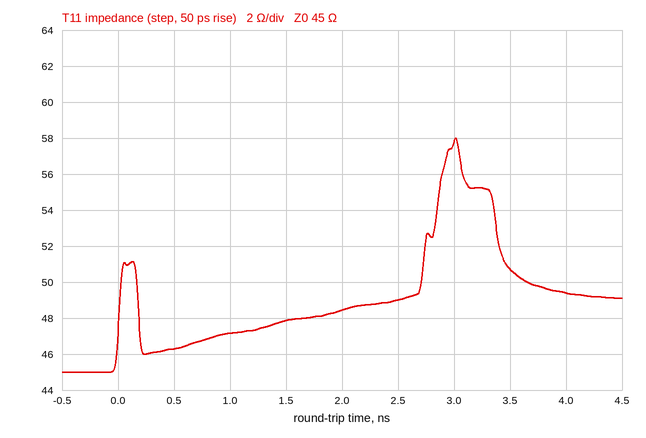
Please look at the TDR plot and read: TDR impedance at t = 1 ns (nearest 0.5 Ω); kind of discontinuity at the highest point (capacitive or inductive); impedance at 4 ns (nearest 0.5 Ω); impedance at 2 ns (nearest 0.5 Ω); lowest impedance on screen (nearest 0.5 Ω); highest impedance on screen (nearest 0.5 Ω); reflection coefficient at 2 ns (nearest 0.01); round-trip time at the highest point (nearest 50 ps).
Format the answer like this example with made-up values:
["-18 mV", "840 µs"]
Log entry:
["47.0 Ω", "inductive", "49.5 Ω", "48.5 Ω", "45.0 Ω", "58.0 Ω", "+0.04", "3.00 ns"]
